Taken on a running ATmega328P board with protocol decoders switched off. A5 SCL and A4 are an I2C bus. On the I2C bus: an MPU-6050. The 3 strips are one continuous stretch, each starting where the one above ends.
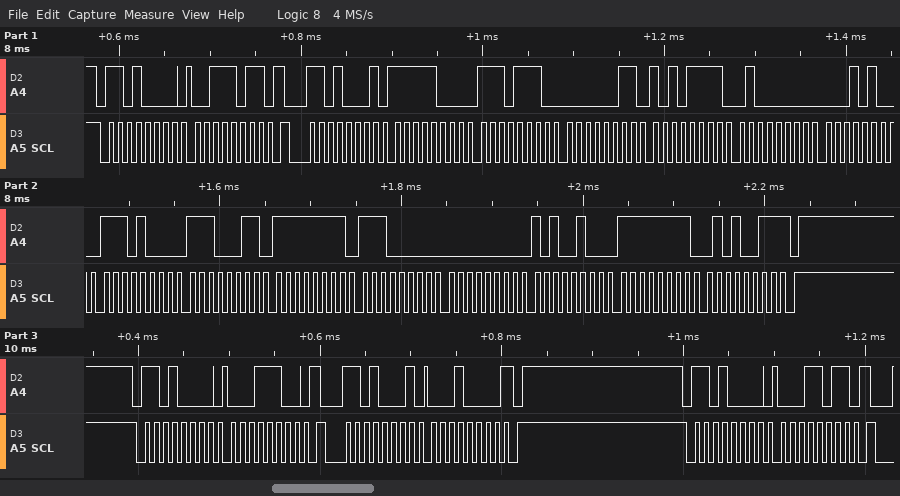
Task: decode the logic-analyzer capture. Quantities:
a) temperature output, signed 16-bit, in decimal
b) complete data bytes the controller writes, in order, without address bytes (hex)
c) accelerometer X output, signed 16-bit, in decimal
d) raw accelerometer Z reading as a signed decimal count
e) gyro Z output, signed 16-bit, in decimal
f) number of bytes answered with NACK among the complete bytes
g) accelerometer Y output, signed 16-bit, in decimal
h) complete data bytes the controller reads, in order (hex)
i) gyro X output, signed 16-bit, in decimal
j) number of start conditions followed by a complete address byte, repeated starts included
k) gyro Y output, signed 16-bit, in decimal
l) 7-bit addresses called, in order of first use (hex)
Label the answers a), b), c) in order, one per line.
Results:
a) -5917
b) 3B 1C 1B
c) -1810
d) 16404
e) -173
f) 2
g) 943
h) F8 EE 03 AF 40 14 E8 E3 FF E0 00 A4 FF 53 10
i) -32
j) 5
k) 164
l) 0x68
